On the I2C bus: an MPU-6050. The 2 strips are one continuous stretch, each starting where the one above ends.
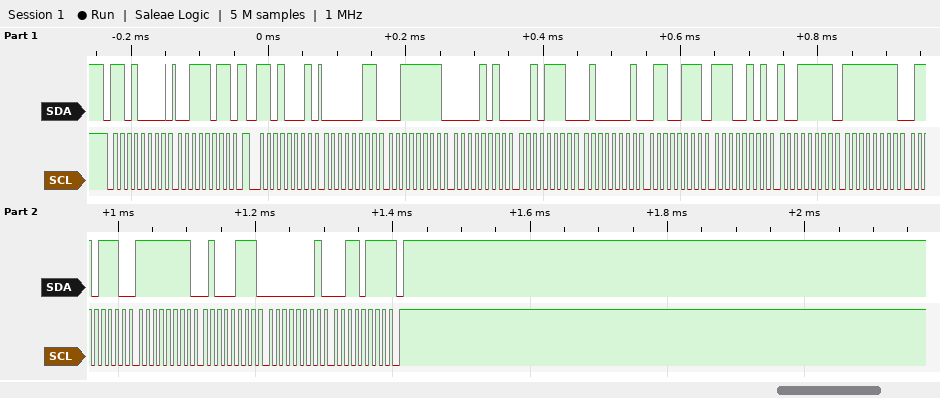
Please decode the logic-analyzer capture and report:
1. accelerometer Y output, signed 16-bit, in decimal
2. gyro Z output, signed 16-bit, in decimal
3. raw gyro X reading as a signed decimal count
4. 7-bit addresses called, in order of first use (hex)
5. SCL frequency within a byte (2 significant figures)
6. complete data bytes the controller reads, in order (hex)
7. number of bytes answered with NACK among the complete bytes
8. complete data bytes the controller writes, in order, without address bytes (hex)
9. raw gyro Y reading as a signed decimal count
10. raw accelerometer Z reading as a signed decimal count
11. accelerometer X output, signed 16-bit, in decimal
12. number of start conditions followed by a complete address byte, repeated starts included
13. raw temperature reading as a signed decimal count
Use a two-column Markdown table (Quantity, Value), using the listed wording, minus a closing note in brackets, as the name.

| Quantity | Value |
|---|---|
| accelerometer Y output, signed 16-bit, in decimal | 2606 |
| gyro Z output, signed 16-bit, in decimal | 311 |
| raw gyro X reading as a signed decimal count | -146 |
| 7-bit addresses called, in order of first use | 0x68 |
| SCL frequency within a byte | 100 kHz |
| complete data bytes the controller reads, in order | 03 3F 0A 2E 41 67 E5 9F FF 6E FF 47 01 37 |
| number of bytes answered with NACK among the complete bytes | 1 |
| complete data bytes the controller writes, in order, without address bytes | 3B |
| raw gyro Y reading as a signed decimal count | -185 |
| raw accelerometer Z reading as a signed decimal count | 16743 |
| accelerometer X output, signed 16-bit, in decimal | 831 |
| number of start conditions followed by a complete address byte, repeated starts included | 2 |
| raw temperature reading as a signed decimal count | -6753 |
